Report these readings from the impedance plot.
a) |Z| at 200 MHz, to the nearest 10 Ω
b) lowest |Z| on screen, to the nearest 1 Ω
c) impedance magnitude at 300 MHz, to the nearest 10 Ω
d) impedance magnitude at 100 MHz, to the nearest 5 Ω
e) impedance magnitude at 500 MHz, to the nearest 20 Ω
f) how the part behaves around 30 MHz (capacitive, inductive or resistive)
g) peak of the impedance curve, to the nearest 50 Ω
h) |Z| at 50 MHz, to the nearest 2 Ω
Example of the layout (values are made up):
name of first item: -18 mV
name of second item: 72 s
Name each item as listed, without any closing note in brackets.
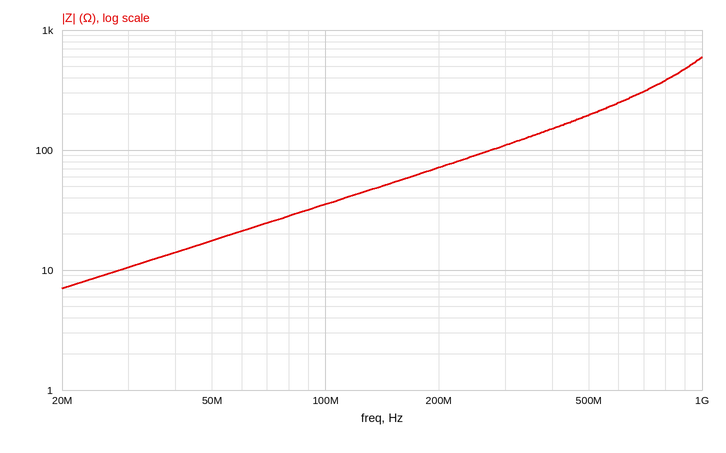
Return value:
|Z| at 200 MHz, to the nearest 10 Ω: 70 Ω
lowest |Z| on screen, to the nearest 1 Ω: 7 Ω
impedance magnitude at 300 MHz, to the nearest 10 Ω: 110 Ω
impedance magnitude at 100 MHz, to the nearest 5 Ω: 35 Ω
impedance magnitude at 500 MHz, to the nearest 20 Ω: 200 Ω
how the part behaves around 30 MHz: inductive
peak of the impedance curve, to the nearest 50 Ω: 600 Ω
|Z| at 50 MHz, to the nearest 2 Ω: 18 Ω
